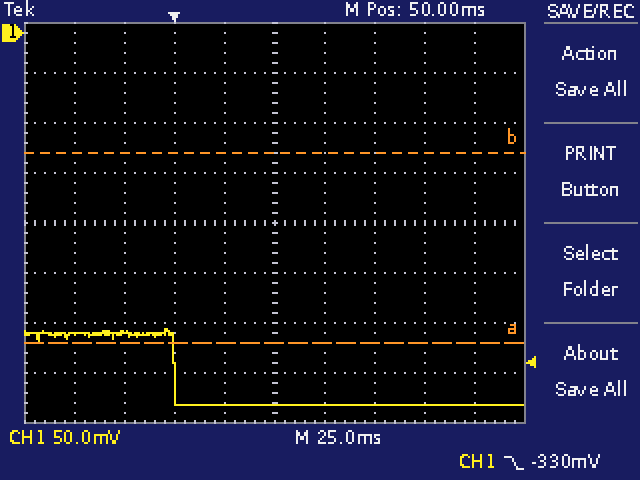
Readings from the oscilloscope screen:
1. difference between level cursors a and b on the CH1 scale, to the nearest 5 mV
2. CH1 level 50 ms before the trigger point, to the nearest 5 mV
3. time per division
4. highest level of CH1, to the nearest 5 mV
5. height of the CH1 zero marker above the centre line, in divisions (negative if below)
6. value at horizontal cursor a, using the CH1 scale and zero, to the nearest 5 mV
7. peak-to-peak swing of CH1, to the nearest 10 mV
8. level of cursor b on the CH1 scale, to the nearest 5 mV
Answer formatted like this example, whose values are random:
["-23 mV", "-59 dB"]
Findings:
["190 mV", "-300 mV", "25 ms", "-295 mV", "+3.8 div", "-310 mV", "80 mV", "-120 mV"]
